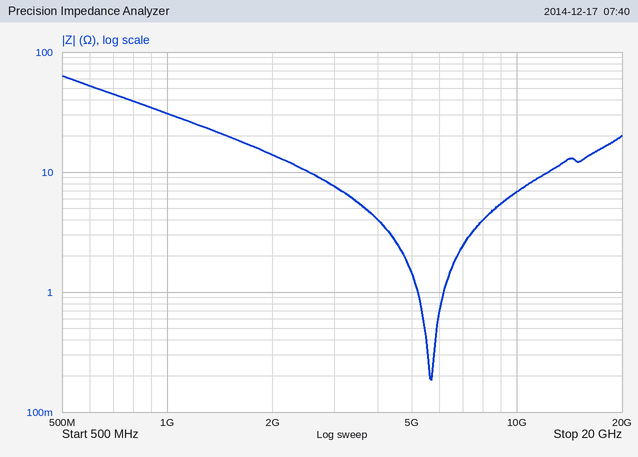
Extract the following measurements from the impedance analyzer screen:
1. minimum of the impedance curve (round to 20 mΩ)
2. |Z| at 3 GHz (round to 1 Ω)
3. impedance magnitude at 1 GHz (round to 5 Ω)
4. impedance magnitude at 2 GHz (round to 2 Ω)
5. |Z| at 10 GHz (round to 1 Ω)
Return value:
180 mΩ
8 Ω
30 Ω
14 Ω
7 Ω
